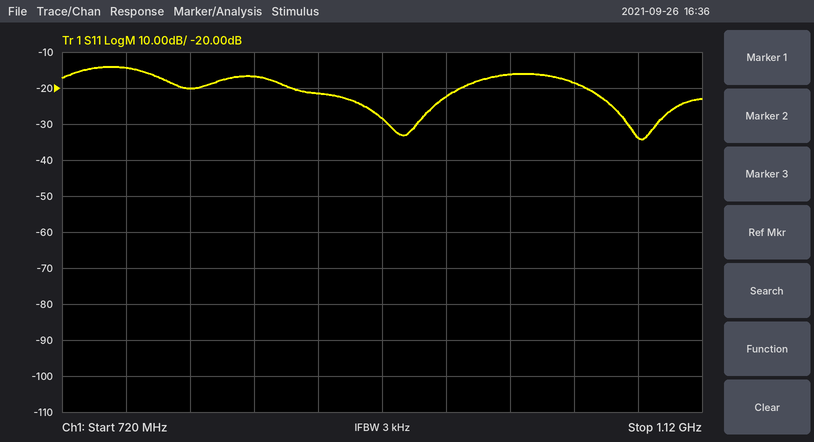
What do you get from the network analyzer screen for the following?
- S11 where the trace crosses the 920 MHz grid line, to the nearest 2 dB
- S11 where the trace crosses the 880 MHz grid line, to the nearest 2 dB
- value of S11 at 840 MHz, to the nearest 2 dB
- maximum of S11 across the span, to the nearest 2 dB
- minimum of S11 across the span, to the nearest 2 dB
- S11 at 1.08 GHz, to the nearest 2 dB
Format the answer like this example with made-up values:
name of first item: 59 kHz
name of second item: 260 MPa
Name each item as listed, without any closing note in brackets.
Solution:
S11 where the trace crosses the 920 MHz grid line, to the nearest 2 dB: -28 dB
S11 where the trace crosses the 880 MHz grid line, to the nearest 2 dB: -22 dB
value of S11 at 840 MHz, to the nearest 2 dB: -16 dB
maximum of S11 across the span, to the nearest 2 dB: -14 dB
minimum of S11 across the span, to the nearest 2 dB: -34 dB
S11 at 1.08 GHz, to the nearest 2 dB: -34 dB
